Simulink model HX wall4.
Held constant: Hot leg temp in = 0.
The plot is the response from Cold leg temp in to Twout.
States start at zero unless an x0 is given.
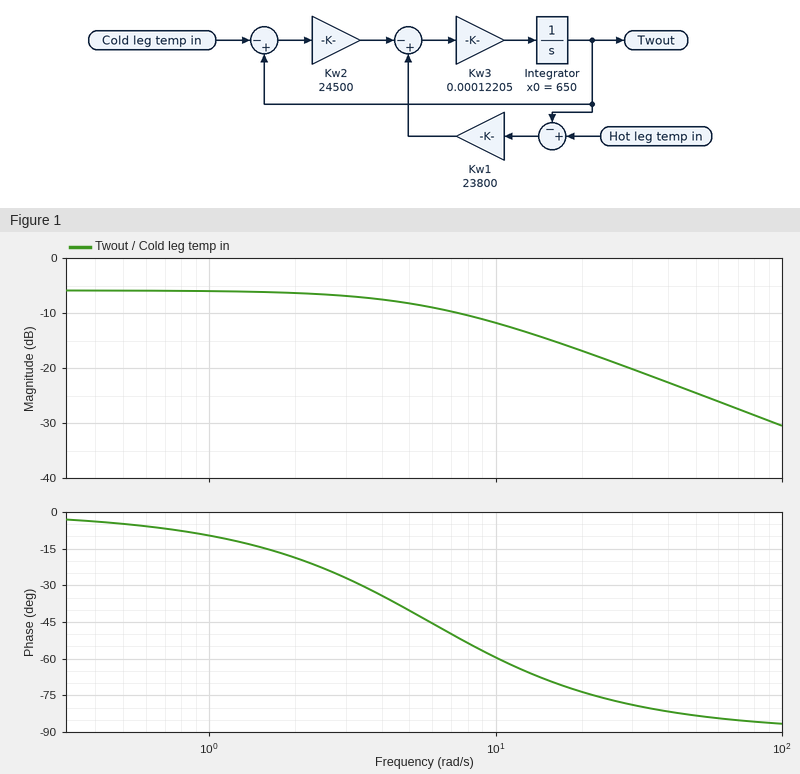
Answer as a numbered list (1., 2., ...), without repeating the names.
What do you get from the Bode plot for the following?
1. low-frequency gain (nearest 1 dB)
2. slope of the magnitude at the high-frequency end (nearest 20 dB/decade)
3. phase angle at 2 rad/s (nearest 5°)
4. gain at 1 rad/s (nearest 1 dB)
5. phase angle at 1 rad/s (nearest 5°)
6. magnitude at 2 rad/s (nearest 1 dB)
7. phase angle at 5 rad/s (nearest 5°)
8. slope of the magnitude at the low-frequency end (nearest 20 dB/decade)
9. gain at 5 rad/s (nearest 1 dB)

1. -6 dB
2. -20 dB/decade
3. -20°
4. -6 dB
5. -10°
6. -6 dB
7. -40°
8. 0 dB/decade
9. -8 dB
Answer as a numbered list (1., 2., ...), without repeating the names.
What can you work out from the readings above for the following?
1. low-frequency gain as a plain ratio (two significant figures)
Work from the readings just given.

1. 0.50
